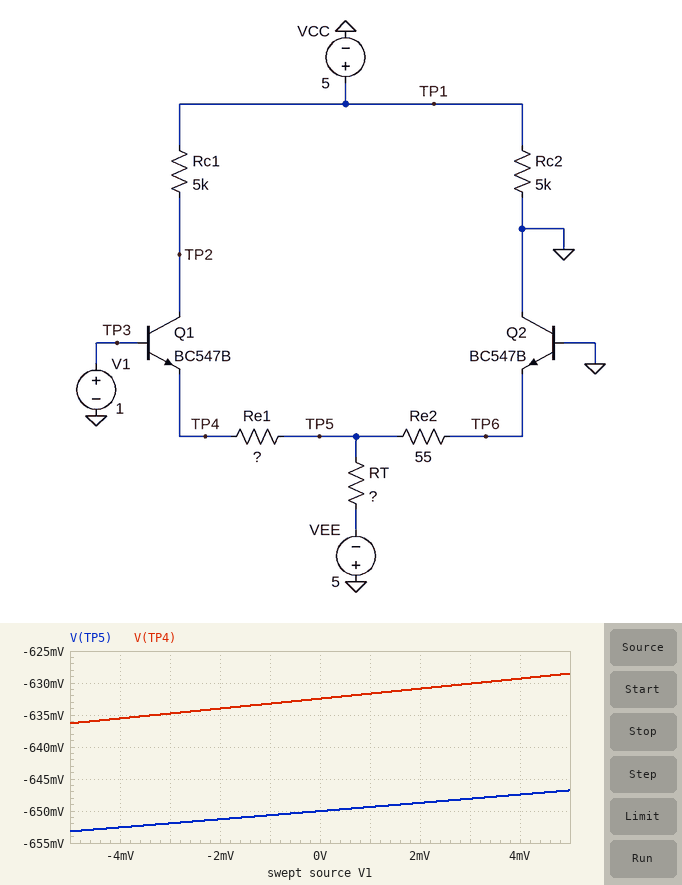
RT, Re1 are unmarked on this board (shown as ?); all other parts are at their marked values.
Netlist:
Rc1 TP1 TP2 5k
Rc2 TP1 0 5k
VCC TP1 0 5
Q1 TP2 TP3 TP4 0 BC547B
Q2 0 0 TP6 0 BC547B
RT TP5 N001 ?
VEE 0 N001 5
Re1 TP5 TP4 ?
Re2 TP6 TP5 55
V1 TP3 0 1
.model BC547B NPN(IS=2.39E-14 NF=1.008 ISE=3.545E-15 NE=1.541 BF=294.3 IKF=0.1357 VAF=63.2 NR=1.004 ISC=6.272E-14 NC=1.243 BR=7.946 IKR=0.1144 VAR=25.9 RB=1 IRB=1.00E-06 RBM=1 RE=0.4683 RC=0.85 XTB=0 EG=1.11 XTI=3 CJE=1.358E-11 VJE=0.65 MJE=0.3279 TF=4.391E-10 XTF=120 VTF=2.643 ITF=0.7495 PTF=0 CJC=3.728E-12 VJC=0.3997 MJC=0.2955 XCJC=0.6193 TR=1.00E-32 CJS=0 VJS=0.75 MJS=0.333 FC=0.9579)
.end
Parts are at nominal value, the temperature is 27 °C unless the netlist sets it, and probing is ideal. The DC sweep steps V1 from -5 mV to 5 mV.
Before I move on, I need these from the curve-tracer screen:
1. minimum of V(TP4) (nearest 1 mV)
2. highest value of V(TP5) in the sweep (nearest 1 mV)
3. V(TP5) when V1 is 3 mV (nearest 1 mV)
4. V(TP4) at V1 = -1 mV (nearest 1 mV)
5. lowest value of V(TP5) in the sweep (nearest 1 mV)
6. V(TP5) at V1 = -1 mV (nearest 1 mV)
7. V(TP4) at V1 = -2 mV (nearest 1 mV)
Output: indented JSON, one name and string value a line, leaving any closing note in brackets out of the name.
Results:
{
  "minimum of V(TP4)": "-636 mV",
  "highest value of V(TP5) in the sweep": "-647 mV",
  "V(TP5) when V1 is 3 mV": "-648 mV",
  "V(TP4) at V1 = -1 mV": "-633 mV",
  "lowest value of V(TP5) in the sweep": "-653 mV",
  "V(TP5) at V1 = -1 mV": "-651 mV",
  "V(TP4) at V1 = -2 mV": "-634 mV"
}
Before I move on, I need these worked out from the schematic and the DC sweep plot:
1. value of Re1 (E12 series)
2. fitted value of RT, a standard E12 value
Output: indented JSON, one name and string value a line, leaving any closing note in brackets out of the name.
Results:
{
  "value of Re1": "22 Ω",
  "fitted value of RT, a standard E12 value": "3.3 kΩ"
}
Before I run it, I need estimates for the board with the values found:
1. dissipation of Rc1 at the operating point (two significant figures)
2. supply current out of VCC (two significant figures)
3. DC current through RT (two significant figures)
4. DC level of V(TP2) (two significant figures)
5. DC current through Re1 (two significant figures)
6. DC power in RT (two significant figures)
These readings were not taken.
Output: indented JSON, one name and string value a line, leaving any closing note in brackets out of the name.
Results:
{
  "dissipation of Rc1 at the operating point": "4.4 mW",
  "supply current out of VCC": "1.9 mA",
  "DC current through RT": "1.6 mA",
  "DC level of V(TP2)": "330 mV",
  "DC current through Re1": "1.6 mA",
  "DC power in RT": "8.4 mW"
}
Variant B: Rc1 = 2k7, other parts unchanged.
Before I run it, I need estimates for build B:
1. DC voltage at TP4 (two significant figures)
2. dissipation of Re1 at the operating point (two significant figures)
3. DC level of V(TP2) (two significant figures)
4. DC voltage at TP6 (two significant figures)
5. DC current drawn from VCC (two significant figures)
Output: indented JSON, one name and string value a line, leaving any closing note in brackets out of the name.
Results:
{
  "DC voltage at TP4": "350 mV",
  "dissipation of Re1 at the operating point": "57 µW",
  "DC level of V(TP2)": "670 mV",
  "DC voltage at TP6": "310 mV",
  "DC current drawn from VCC": "2.6 mA"
}
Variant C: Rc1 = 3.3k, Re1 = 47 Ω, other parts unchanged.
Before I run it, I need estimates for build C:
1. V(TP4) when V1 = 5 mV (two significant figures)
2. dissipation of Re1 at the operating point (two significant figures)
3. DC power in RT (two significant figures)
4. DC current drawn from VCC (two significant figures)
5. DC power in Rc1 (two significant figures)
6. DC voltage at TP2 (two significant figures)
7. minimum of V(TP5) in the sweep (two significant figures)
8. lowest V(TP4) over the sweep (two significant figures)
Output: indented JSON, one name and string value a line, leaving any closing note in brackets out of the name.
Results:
{
  "V(TP4) when V1 = 5 mV": "-620 mV",
  "dissipation of Re1 at the operating point": "120 µW",
  "DC power in RT": "8.4 mW",
  "DC current drawn from VCC": "2.4 mA",
  "DC power in Rc1": "6.5 mW",
  "DC voltage at TP2": "360 mV",
  "minimum of V(TP5) in the sweep": "-660 mV",
  "lowest V(TP4) over the sweep": "-630 mV"
}
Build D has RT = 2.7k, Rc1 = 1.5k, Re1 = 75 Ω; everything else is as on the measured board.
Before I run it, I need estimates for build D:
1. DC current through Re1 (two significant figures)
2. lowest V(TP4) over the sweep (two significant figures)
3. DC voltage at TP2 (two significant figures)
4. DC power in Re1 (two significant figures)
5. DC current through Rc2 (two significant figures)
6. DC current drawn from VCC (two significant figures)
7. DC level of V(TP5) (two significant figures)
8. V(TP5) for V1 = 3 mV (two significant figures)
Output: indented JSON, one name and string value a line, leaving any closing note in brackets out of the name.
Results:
{
  "DC current through Re1": "1.9 mA",
  "lowest V(TP4) over the sweep": "-630 mV",
  "DC voltage at TP2": "2.1 V",
  "DC power in Re1": "280 µW",
  "DC current through Rc2": "1.0 mA",
  "DC current drawn from VCC": "2.9 mA",
  "DC level of V(TP5)": "200 mV",
  "V(TP5) for V1 = 3 mV": "-680 mV"
}
